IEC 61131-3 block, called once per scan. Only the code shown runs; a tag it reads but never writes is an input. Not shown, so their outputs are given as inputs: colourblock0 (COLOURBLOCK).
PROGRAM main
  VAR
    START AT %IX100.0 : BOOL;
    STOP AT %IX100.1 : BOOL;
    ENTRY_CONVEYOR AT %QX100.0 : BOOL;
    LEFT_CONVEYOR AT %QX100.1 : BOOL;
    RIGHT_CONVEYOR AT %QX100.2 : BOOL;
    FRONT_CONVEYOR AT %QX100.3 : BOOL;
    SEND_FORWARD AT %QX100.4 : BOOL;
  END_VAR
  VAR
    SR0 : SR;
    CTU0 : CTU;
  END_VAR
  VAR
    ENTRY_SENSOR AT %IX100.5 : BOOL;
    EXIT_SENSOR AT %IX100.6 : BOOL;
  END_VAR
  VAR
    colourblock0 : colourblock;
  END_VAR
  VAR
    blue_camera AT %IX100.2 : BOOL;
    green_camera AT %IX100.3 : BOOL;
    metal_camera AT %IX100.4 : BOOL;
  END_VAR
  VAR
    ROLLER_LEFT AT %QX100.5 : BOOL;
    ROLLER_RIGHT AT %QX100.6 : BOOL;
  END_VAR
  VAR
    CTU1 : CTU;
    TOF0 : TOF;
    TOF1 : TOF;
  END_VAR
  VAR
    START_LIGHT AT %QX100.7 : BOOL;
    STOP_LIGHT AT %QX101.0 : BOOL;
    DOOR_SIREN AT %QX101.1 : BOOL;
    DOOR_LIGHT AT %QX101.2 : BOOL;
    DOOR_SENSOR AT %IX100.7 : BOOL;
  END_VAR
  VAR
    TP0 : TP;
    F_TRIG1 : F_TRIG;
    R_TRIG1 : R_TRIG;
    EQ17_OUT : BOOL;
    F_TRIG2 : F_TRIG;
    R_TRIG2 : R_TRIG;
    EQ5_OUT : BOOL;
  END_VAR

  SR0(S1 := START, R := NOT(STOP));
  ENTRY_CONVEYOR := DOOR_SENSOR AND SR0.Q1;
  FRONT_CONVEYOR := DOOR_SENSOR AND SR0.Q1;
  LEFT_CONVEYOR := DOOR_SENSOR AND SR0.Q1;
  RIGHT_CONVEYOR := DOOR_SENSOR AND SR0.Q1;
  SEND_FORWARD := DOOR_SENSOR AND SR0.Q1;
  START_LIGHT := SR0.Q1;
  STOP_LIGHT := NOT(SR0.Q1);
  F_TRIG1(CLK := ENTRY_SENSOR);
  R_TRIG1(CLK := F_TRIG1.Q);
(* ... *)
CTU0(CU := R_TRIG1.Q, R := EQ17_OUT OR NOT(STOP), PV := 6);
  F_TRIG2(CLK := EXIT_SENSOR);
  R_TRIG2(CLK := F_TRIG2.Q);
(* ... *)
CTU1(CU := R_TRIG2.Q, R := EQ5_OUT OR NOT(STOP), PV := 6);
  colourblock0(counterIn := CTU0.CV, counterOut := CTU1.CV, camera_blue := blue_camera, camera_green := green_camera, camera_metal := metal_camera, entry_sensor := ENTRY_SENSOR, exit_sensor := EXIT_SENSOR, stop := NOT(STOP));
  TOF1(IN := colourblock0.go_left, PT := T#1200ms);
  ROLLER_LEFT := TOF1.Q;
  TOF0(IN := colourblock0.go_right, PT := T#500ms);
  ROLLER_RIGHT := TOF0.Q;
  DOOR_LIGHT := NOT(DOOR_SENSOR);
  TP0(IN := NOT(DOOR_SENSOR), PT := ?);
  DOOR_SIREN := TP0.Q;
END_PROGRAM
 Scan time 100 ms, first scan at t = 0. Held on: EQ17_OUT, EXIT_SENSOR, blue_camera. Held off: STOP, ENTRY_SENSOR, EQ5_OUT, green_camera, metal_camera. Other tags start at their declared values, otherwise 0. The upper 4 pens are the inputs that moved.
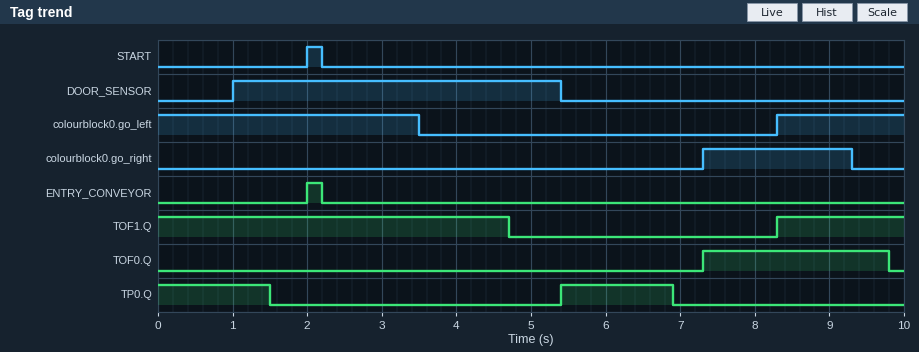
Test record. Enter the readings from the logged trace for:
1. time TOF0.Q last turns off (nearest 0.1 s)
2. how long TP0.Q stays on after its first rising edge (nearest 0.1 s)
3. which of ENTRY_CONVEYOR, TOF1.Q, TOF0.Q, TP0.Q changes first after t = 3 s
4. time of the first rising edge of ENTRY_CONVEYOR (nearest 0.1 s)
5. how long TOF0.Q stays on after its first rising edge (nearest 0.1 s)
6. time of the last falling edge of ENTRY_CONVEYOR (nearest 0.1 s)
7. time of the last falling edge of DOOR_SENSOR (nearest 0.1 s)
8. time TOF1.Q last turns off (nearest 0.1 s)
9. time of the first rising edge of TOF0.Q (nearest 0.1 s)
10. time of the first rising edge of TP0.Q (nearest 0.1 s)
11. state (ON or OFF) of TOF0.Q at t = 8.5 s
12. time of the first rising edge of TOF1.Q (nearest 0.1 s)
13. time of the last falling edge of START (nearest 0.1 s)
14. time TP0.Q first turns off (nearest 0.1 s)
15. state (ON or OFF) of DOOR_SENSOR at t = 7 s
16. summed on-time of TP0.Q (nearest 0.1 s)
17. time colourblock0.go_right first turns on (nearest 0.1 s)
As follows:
9.8 s
1.5 s
TOF1.Q
2.0 s
2.5 s
2.2 s
5.4 s
4.7 s
7.3 s
5.4 s
ON
8.3 s
2.2 s
1.5 s
OFF
3.0 s
7.3 s
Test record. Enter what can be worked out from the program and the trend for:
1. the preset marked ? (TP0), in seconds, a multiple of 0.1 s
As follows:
1.5 s
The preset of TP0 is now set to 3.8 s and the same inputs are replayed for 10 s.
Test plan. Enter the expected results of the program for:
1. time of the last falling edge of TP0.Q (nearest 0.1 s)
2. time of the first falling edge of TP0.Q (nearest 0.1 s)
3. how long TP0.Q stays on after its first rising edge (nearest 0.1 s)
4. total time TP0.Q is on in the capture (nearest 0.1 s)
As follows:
9.2 s
3.8 s
3.8 s
7.6 s
